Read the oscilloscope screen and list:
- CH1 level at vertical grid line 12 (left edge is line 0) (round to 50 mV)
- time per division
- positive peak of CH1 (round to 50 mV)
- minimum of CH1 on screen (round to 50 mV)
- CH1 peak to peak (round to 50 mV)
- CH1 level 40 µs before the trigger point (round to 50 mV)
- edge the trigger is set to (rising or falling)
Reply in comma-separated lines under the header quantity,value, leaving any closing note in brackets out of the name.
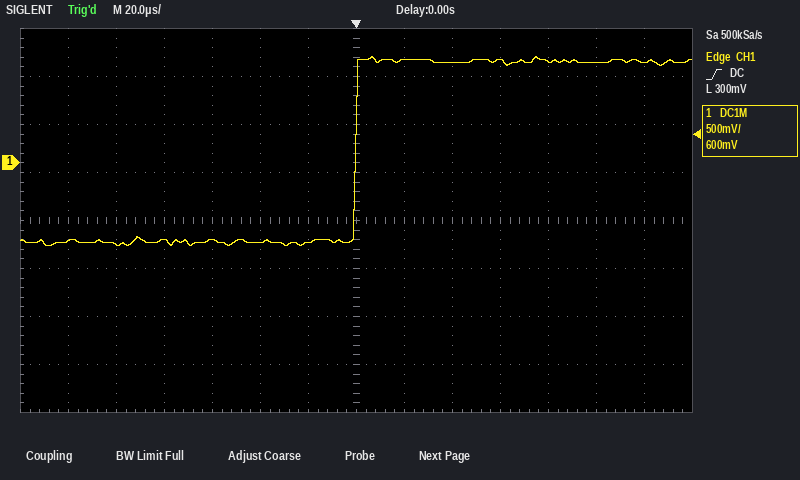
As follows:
quantity,value
CH1 level at vertical grid line 12 (left edge is line 0),1.05 V
time per division,20 µs
positive peak of CH1,1.10 V
minimum of CH1 on screen,-850 mV
CH1 peak to peak,1.95 V
CH1 level 40 µs before the trigger point,-850 mV
edge the trigger is set to,rising
